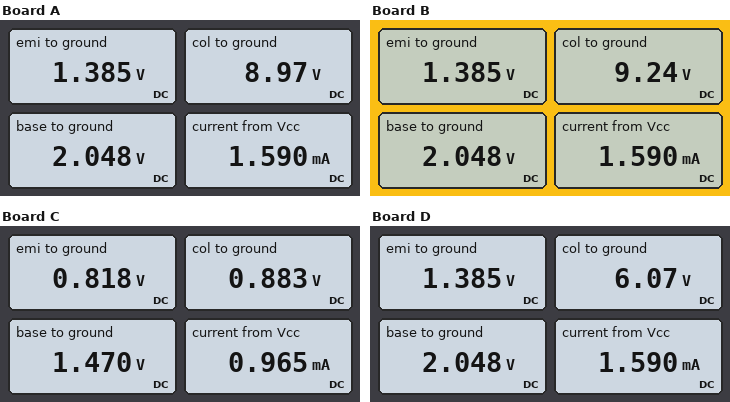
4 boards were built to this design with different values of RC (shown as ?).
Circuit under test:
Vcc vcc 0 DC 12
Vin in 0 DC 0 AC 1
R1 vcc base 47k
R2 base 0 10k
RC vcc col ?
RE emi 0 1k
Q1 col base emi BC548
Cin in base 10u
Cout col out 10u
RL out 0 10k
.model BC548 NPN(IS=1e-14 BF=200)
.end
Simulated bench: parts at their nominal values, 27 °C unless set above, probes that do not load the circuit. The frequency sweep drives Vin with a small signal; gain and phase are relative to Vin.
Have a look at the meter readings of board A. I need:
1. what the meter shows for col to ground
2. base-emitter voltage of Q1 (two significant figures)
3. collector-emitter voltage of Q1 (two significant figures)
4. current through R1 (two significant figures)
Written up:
8.97 V
660 mV
7.6 V
210 µA
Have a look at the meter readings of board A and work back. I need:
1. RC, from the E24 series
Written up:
2.2 kΩ
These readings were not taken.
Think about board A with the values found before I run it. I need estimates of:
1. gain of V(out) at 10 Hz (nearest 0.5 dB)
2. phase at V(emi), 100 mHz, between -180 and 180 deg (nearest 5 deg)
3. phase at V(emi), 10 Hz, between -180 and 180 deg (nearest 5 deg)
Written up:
4.5 dB
85 deg
10 deg
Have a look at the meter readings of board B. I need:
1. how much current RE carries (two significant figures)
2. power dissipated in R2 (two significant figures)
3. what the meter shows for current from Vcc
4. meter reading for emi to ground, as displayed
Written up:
1.4 mA
420 µW
1.590 mA
1.385 V
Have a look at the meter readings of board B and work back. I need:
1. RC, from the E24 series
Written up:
2 kΩ
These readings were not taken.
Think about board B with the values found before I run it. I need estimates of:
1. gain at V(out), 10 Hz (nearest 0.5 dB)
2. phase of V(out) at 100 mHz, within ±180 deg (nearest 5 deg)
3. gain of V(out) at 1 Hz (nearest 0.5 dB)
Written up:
4.0 dB
-5 deg
-7.0 dB
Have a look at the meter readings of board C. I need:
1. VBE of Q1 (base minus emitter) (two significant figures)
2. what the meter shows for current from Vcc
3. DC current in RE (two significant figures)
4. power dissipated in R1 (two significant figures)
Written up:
650 mV
0.965 mA
820 µA
2.4 mW
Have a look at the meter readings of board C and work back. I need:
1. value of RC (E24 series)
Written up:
15 kΩ
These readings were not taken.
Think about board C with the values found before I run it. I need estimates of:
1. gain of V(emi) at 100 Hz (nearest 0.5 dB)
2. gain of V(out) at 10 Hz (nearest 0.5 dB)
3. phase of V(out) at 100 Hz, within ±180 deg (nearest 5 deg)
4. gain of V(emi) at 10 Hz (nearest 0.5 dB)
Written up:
-0.5 dB
-10.5 dB
10 deg
-7.0 dB
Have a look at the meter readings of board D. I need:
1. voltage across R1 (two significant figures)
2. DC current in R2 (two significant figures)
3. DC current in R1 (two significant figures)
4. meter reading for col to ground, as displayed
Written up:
10 V
200 µA
210 µA
6.07 V
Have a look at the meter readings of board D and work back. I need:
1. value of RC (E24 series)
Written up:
4.3 kΩ
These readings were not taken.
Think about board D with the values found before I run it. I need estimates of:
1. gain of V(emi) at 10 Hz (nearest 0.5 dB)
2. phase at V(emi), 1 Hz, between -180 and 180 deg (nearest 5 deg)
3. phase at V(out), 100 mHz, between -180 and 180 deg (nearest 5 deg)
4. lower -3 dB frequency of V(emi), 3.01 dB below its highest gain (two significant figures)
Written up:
-0.5 dB
65 deg
-10 deg
2.0 Hz
